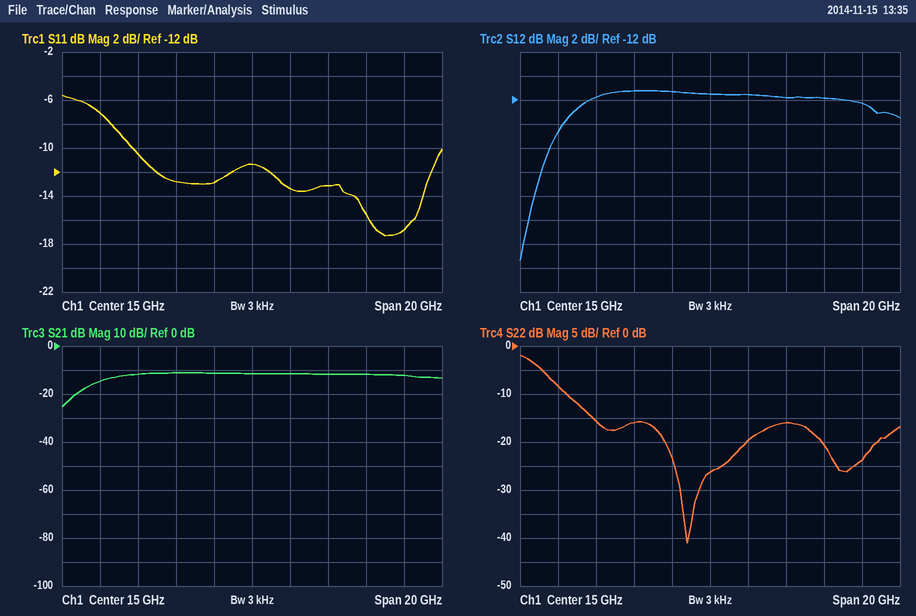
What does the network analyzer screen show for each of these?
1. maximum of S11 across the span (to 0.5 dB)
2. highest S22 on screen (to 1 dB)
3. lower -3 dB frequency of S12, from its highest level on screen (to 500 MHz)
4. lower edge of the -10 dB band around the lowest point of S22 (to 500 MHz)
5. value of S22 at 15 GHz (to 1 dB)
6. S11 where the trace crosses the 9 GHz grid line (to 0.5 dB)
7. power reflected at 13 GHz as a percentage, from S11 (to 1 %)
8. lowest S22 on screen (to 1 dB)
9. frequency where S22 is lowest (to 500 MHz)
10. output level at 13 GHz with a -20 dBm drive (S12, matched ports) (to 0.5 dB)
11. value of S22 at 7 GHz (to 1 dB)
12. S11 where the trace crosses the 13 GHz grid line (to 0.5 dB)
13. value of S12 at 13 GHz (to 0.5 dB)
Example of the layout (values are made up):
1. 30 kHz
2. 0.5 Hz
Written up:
1. -5.5 dB
2. -2 dB
3. 7.0 GHz
4. 7.5 GHz
5. -26 dB
6. -10.5 dB
7. 5 %
8. -41 dB
9. 14.0 GHz
10. -31.5 dBm
11. -8 dB
12. -13.0 dB
13. -11.5 dB
